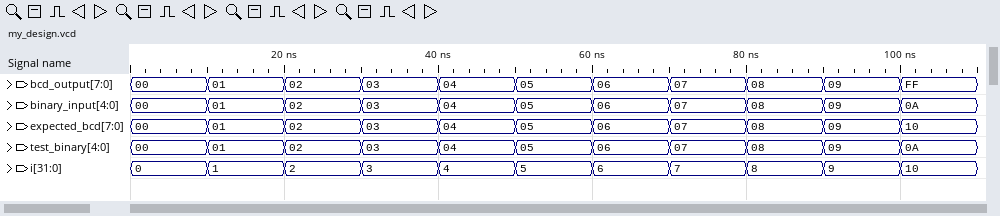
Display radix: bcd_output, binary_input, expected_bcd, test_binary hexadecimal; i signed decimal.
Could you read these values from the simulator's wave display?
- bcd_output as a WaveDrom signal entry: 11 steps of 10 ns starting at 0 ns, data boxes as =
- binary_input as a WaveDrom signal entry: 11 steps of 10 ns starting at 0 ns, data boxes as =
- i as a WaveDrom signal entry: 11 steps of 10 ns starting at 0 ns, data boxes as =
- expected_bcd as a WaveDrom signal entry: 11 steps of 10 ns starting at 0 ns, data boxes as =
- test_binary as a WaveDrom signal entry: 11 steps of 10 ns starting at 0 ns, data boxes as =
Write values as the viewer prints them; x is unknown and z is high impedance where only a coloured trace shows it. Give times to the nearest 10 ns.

{name: 'bcd_output', wave: '===========', data: '00 01 02 03 04 05 06 07 08 09 FF'}
{name: 'binary_input', wave: '===========', data: '00 01 02 03 04 05 06 07 08 09 0A'}
{name: 'i', wave: '===========', data: '0 1 2 3 4 5 6 7 8 9 10'}
{name: 'expected_bcd', wave: '===========', data: '00 01 02 03 04 05 06 07 08 09 10'}
{name: 'test_binary', wave: '===========', data: '00 01 02 03 04 05 06 07 08 09 0A'}
